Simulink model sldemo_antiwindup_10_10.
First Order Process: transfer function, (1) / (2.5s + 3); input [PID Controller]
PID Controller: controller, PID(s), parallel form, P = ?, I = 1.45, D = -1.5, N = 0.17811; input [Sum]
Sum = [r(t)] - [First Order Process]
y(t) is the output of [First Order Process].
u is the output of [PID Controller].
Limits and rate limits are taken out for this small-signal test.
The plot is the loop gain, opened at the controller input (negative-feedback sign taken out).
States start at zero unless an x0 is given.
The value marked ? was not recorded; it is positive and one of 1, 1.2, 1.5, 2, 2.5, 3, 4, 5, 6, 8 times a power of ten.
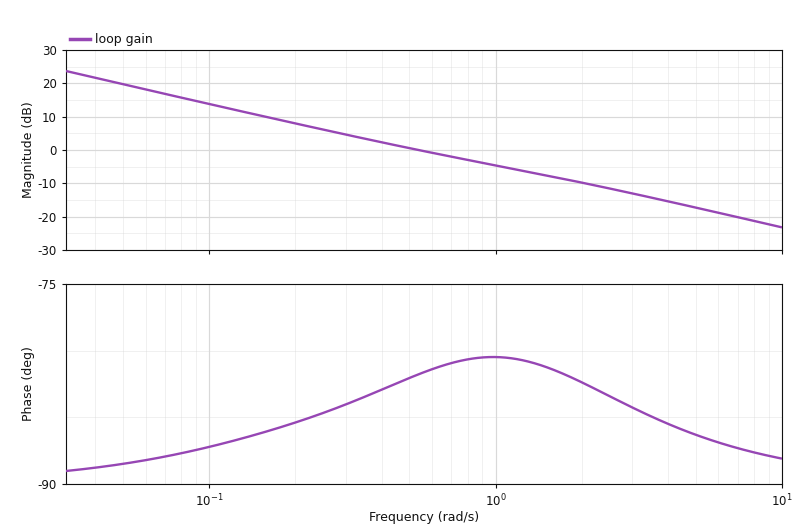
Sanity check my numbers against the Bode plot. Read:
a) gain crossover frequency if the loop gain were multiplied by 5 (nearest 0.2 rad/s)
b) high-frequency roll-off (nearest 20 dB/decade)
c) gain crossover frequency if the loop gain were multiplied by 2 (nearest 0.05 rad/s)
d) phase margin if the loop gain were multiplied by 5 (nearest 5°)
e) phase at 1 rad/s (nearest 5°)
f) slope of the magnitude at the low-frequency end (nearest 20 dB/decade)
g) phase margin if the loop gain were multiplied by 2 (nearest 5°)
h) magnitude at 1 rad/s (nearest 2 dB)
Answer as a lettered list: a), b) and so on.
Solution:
a) 3.4 rad/s
b) -20 dB/decade
c) 1.20 rad/s
d) 95°
e) -80°
f) -20 dB/decade
g) 100°
h) -4 dB
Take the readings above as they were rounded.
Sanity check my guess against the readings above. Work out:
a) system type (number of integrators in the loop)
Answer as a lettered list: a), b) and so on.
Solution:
a) 1
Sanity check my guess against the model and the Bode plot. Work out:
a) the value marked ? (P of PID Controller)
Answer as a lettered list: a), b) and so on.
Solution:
a) 2
